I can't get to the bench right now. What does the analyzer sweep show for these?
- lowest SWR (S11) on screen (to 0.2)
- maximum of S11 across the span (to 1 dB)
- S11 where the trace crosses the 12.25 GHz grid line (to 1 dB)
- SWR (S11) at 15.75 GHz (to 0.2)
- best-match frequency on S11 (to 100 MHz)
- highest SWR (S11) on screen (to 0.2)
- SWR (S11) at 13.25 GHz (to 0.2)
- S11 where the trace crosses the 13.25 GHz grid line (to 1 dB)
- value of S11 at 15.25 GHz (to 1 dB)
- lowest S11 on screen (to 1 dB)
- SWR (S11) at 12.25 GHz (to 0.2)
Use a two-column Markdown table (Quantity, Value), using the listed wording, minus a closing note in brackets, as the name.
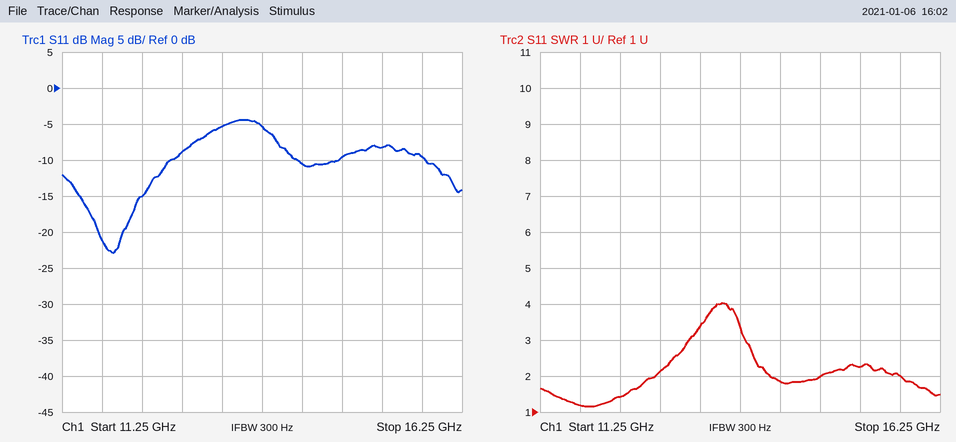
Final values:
| Quantity | Value |
|---|---|
| lowest SWR (S11) on screen | 1.2 |
| maximum of S11 across the span | -4 dB |
| S11 where the trace crosses the 12.25 GHz grid line | -15 dB |
| SWR (S11) at 15.75 GHz | 2.0 |
| best-match frequency on S11 | 11.9 GHz |
| highest SWR (S11) on screen | 4.0 |
| SWR (S11) at 13.25 GHz | 3.4 |
| S11 where the trace crosses the 13.25 GHz grid line | -5 dB |
| value of S11 at 15.25 GHz | -8 dB |
| lowest S11 on screen | -23 dB |
| SWR (S11) at 12.25 GHz | 1.4 |
